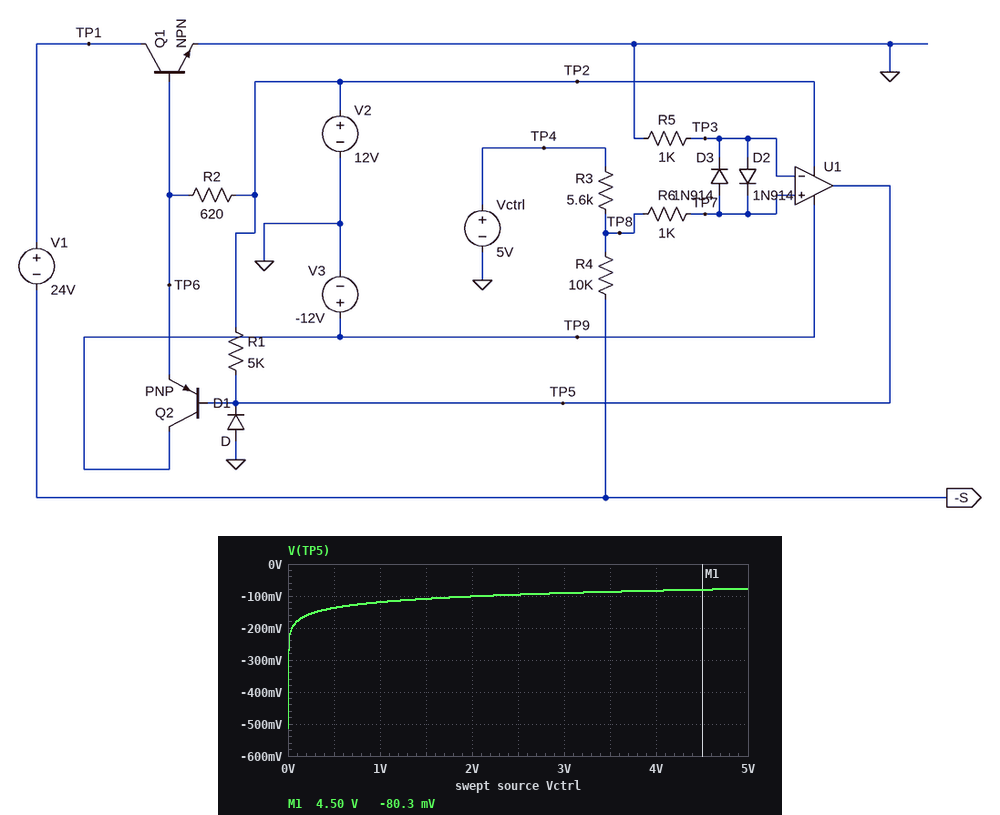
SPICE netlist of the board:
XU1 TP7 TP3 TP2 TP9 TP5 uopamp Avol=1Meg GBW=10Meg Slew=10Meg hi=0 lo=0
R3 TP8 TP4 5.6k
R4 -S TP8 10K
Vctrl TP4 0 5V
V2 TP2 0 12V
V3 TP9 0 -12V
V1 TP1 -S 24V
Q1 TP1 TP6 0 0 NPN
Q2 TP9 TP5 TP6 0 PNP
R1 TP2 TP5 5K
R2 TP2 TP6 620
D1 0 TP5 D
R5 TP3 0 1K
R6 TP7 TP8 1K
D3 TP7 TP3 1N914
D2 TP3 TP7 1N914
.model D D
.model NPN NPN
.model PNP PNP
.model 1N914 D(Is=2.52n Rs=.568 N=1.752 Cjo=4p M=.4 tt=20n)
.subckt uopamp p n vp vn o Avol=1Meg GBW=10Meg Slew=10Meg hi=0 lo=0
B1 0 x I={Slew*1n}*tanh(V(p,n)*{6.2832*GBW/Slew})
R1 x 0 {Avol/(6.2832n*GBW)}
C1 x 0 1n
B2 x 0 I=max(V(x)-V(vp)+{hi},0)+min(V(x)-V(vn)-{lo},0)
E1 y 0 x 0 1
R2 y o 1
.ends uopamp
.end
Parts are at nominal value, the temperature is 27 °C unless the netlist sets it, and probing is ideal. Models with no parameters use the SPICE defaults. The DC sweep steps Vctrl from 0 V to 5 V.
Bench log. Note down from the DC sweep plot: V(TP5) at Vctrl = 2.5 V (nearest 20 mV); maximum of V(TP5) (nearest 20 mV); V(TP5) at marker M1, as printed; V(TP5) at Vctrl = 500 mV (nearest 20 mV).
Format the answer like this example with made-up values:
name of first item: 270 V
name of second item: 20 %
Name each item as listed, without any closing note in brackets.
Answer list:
V(TP5) at Vctrl = 2.5 V: -100 mV
maximum of V(TP5): -80 mV
V(TP5) at marker M1, as printed: -80.3 mV
V(TP5) at Vctrl = 500 mV: -140 mV
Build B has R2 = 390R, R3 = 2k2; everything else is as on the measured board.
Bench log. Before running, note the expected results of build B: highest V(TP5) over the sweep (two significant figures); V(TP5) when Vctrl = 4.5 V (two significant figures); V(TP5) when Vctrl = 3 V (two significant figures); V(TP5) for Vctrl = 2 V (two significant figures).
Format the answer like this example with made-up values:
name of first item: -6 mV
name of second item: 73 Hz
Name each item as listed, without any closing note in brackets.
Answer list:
highest V(TP5) over the sweep: -65 mV
V(TP5) when Vctrl = 4.5 V: -68 mV
V(TP5) when Vctrl = 3 V: -79 mV
V(TP5) for Vctrl = 2 V: -89 mV
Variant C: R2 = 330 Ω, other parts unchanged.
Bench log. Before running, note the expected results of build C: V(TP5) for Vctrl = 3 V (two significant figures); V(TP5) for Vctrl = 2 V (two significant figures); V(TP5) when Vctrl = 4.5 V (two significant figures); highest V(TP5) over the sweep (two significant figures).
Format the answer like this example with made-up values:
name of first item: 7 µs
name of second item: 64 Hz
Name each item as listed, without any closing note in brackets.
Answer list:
V(TP5) for Vctrl = 3 V: -110 mV
V(TP5) for Vctrl = 2 V: -120 mV
V(TP5) when Vctrl = 4.5 V: -97 mV
highest V(TP5) over the sweep: -94 mV
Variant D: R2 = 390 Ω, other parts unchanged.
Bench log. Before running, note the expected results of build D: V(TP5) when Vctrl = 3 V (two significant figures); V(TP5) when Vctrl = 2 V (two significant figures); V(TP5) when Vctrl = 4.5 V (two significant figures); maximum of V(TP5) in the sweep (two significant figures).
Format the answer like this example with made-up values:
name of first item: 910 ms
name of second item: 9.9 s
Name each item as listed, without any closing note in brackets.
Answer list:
V(TP5) when Vctrl = 3 V: -100 mV
V(TP5) when Vctrl = 2 V: -110 mV
V(TP5) when Vctrl = 4.5 V: -92 mV
maximum of V(TP5) in the sweep: -90 mV
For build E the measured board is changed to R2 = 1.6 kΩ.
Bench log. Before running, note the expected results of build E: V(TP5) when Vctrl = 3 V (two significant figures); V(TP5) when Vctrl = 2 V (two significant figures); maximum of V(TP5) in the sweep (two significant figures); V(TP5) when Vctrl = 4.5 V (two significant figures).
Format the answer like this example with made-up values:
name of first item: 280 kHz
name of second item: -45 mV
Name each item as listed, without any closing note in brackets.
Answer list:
V(TP5) when Vctrl = 3 V: -66 mV
V(TP5) when Vctrl = 2 V: -77 mV
maximum of V(TP5) in the sweep: -53 mV
V(TP5) when Vctrl = 4.5 V: -56 mV
